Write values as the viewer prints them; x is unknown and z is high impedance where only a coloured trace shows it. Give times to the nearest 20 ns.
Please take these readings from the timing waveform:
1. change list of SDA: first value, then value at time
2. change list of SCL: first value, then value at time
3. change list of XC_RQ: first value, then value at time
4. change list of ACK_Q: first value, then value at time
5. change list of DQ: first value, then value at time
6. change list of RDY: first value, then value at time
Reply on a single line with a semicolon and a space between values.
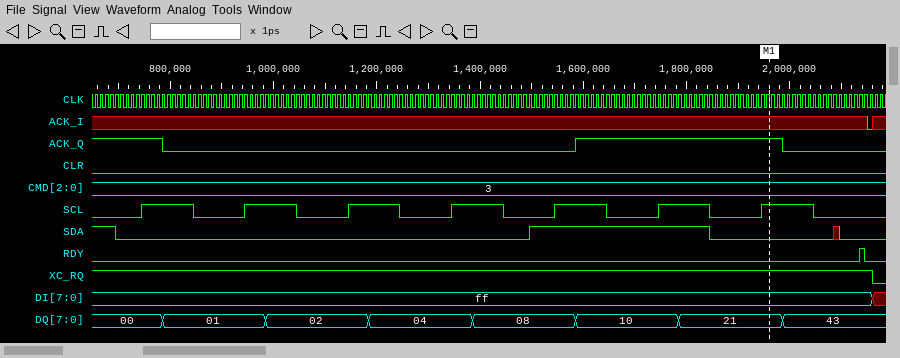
1, 0 at 700 ns, 1 at 1500 ns, 0 at 1840 ns, x at 2080 ns, 0 at 2100 ns; 0, 1 at 740 ns, 0 at 840 ns, 1 at 940 ns, 0 at 1040 ns, 1 at 1140 ns, 0 at 1240 ns, 1 at 1340 ns, 0 at 1440 ns, 1 at 1540 ns, 0 at 1640 ns, 1 at 1740 ns, 0 at 1840 ns, 1 at 1940 ns, 0 at 2040 ns; 1, 0 at 2160 ns; 1, 0 at 780 ns, 1 at 1580 ns, 0 at 1980 ns; 00, 01 at 780 ns, 02 at 980 ns, 04 at 1180 ns, 08 at 1380 ns, 10 at 1580 ns, 21 at 1780 ns, 43 at 1980 ns; 0, 1 at 2140 ns, 0 at 2140 ns
